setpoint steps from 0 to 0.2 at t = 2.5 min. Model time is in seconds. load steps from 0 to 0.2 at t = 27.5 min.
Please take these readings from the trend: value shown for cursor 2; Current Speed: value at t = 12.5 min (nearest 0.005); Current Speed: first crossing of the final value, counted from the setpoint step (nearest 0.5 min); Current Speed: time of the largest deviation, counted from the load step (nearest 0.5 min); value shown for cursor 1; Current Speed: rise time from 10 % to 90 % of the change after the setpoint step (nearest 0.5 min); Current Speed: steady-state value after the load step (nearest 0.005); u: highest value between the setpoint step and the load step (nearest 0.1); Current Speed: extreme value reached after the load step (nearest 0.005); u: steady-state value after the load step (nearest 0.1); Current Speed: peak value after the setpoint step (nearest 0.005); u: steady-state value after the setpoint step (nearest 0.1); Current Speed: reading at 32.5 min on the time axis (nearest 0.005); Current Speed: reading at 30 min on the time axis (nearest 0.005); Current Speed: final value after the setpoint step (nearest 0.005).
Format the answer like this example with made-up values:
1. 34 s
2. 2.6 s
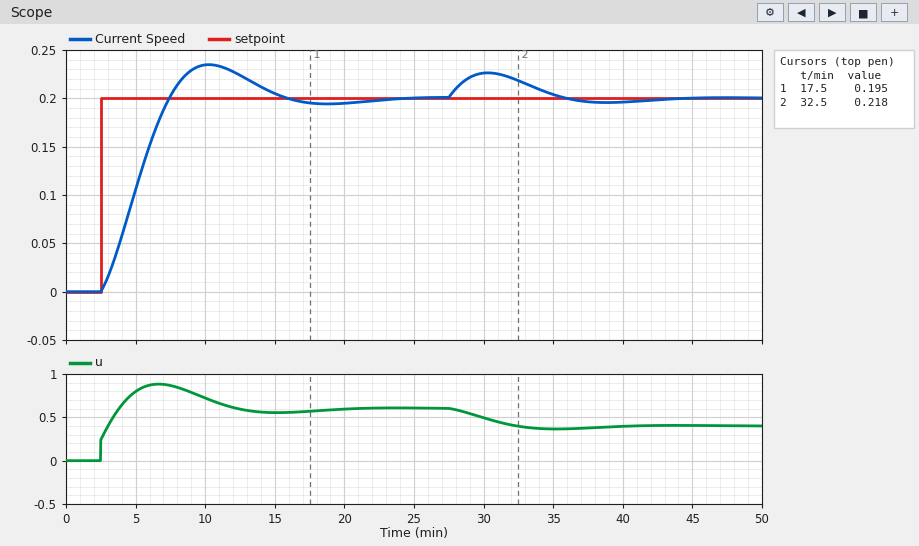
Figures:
1. 0.218
2. 0.225
3. 5.0 min
4. 3.0 min
5. 0.195
6. 3.5 min
7. 0.200
8. 0.9
9. 0.225
10. 0.4
11. 0.235
12. 0.6
13. 0.220
14. 0.225
15. 0.200
